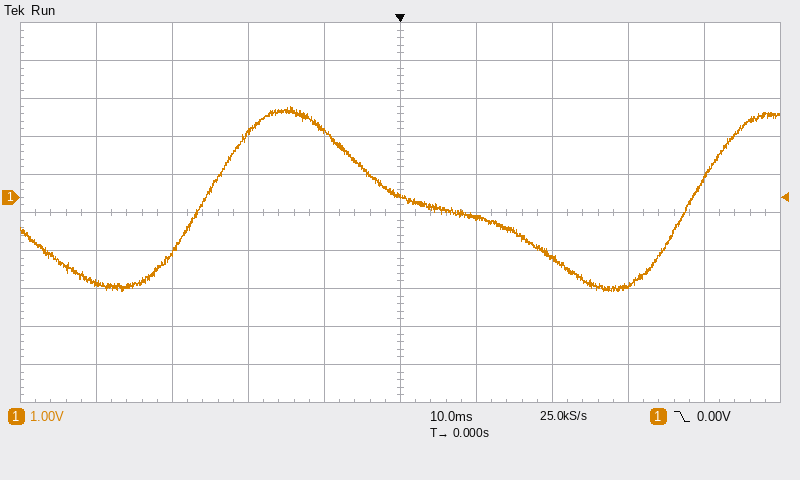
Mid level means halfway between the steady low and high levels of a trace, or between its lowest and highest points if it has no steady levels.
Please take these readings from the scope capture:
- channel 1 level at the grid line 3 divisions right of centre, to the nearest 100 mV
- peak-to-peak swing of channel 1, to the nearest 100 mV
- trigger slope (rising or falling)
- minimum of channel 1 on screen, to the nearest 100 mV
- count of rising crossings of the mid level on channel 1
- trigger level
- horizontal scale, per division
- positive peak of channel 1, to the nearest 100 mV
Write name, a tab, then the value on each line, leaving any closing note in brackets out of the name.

channel 1 level at the grid line 3 divisions right of centre, to the nearest 100 mV	-2.3 V
peak-to-peak swing of channel 1, to the nearest 100 mV	4.9 V
trigger slope	falling
minimum of channel 1 on screen, to the nearest 100 mV	-2.5 V
count of rising crossings of the mid level on channel 1	2
trigger level	0.00 V
horizontal scale, per division	10 ms
positive peak of channel 1, to the nearest 100 mV	2.4 V
